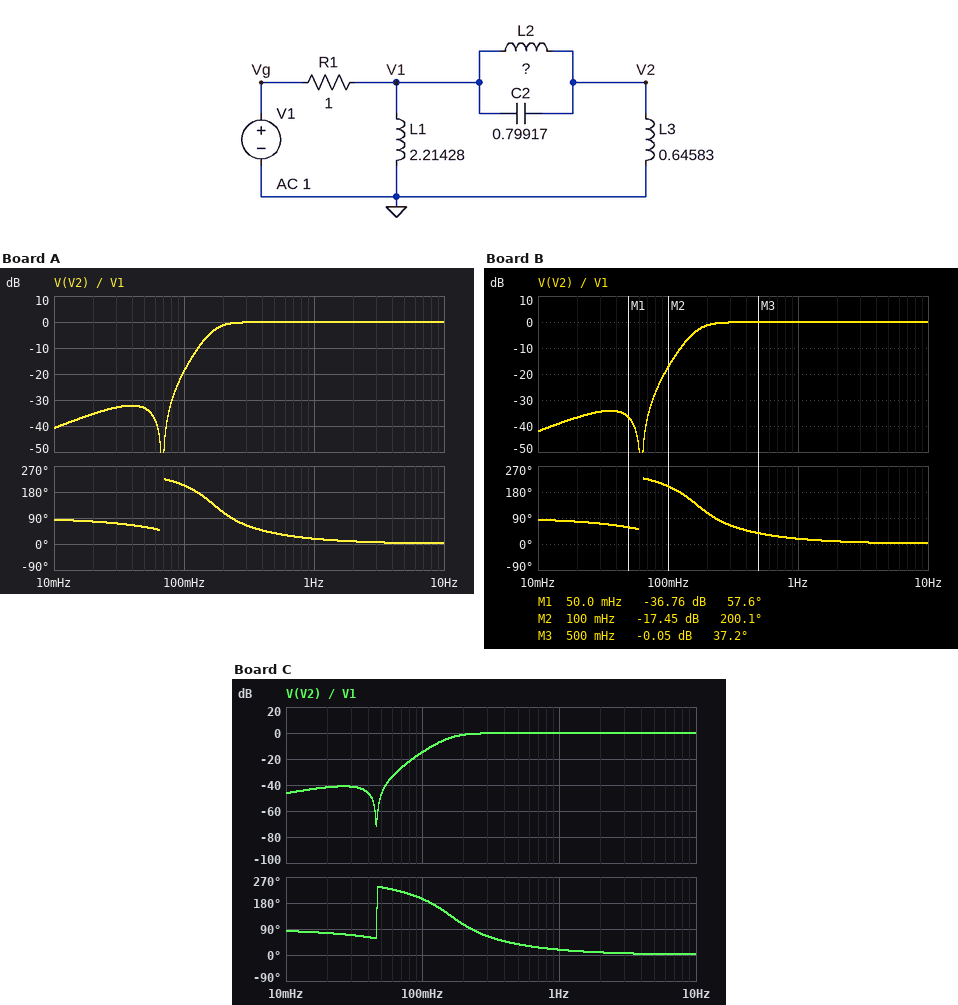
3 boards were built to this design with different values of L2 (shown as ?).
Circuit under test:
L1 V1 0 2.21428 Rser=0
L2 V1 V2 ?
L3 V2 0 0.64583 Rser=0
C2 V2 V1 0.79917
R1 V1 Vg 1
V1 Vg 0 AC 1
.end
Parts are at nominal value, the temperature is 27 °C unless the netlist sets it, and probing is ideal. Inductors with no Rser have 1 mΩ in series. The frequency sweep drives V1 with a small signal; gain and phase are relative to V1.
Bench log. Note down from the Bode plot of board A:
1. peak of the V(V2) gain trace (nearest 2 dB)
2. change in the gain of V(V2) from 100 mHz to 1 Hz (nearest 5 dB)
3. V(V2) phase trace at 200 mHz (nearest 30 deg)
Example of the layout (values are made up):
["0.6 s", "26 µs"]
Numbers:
["0 dB", "20 dB", "120 deg"]
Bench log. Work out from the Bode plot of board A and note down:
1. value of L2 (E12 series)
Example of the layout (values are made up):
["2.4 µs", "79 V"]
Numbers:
["6.8 H"]
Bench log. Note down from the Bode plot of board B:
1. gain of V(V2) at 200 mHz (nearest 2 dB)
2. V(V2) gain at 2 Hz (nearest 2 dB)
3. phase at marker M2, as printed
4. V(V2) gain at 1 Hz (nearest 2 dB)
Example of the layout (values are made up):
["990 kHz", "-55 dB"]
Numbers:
["-2 dB", "0 dB", "200.1 deg", "0 dB"]
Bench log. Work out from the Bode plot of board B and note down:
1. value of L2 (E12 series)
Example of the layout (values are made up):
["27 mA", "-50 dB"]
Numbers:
["8.2 H"]
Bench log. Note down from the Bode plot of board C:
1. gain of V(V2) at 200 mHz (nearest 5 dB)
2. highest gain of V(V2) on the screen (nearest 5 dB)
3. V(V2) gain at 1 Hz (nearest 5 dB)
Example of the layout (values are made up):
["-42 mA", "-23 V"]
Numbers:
["0 dB", "0 dB", "0 dB"]
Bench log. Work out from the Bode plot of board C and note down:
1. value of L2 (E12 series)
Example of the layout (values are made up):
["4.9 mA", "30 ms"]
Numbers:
["15 H"]
